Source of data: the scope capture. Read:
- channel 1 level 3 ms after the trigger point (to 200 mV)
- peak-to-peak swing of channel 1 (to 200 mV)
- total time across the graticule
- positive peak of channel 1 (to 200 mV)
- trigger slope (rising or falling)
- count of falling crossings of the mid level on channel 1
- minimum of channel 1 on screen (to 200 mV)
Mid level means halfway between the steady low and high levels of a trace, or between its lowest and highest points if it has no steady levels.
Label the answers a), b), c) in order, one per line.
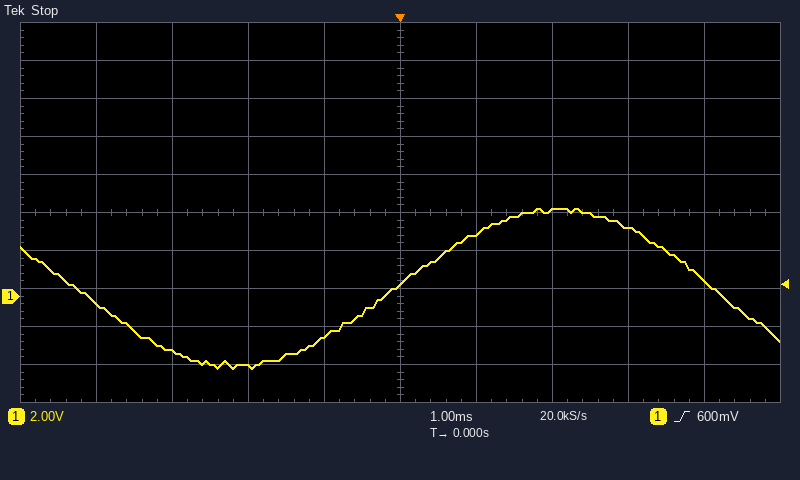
a) 3.6 V
b) 8.4 V
c) 10 ms
d) 4.6 V
e) rising
f) 2
g) -3.8 V
